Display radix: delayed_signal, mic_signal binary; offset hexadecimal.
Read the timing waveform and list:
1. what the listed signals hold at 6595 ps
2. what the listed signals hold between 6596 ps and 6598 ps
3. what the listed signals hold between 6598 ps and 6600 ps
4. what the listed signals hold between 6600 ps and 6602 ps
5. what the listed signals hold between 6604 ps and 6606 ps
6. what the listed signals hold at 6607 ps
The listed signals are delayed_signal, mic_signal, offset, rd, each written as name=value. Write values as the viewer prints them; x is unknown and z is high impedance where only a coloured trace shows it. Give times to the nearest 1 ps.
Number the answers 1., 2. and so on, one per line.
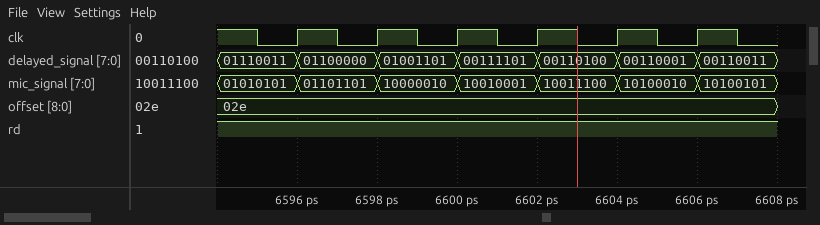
1. delayed_signal=01110011, mic_signal=01010101, offset=02e, rd=1
2. delayed_signal=01100000, mic_signal=01101101, offset=02e, rd=1
3. delayed_signal=01001101, mic_signal=10000010, offset=02e, rd=1
4. delayed_signal=00111101, mic_signal=10010001, offset=02e, rd=1
5. delayed_signal=00110001, mic_signal=10100010, offset=02e, rd=1
6. delayed_signal=00110011, mic_signal=10100101, offset=02e, rd=1
